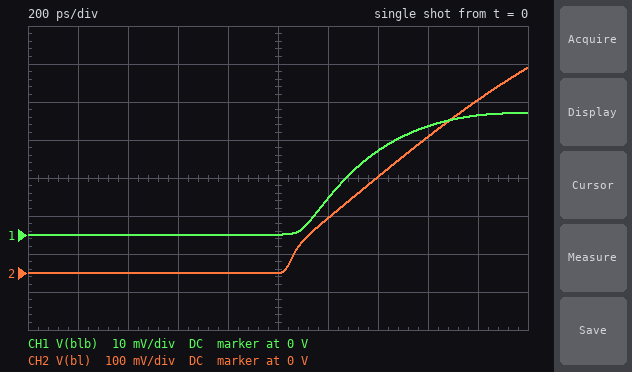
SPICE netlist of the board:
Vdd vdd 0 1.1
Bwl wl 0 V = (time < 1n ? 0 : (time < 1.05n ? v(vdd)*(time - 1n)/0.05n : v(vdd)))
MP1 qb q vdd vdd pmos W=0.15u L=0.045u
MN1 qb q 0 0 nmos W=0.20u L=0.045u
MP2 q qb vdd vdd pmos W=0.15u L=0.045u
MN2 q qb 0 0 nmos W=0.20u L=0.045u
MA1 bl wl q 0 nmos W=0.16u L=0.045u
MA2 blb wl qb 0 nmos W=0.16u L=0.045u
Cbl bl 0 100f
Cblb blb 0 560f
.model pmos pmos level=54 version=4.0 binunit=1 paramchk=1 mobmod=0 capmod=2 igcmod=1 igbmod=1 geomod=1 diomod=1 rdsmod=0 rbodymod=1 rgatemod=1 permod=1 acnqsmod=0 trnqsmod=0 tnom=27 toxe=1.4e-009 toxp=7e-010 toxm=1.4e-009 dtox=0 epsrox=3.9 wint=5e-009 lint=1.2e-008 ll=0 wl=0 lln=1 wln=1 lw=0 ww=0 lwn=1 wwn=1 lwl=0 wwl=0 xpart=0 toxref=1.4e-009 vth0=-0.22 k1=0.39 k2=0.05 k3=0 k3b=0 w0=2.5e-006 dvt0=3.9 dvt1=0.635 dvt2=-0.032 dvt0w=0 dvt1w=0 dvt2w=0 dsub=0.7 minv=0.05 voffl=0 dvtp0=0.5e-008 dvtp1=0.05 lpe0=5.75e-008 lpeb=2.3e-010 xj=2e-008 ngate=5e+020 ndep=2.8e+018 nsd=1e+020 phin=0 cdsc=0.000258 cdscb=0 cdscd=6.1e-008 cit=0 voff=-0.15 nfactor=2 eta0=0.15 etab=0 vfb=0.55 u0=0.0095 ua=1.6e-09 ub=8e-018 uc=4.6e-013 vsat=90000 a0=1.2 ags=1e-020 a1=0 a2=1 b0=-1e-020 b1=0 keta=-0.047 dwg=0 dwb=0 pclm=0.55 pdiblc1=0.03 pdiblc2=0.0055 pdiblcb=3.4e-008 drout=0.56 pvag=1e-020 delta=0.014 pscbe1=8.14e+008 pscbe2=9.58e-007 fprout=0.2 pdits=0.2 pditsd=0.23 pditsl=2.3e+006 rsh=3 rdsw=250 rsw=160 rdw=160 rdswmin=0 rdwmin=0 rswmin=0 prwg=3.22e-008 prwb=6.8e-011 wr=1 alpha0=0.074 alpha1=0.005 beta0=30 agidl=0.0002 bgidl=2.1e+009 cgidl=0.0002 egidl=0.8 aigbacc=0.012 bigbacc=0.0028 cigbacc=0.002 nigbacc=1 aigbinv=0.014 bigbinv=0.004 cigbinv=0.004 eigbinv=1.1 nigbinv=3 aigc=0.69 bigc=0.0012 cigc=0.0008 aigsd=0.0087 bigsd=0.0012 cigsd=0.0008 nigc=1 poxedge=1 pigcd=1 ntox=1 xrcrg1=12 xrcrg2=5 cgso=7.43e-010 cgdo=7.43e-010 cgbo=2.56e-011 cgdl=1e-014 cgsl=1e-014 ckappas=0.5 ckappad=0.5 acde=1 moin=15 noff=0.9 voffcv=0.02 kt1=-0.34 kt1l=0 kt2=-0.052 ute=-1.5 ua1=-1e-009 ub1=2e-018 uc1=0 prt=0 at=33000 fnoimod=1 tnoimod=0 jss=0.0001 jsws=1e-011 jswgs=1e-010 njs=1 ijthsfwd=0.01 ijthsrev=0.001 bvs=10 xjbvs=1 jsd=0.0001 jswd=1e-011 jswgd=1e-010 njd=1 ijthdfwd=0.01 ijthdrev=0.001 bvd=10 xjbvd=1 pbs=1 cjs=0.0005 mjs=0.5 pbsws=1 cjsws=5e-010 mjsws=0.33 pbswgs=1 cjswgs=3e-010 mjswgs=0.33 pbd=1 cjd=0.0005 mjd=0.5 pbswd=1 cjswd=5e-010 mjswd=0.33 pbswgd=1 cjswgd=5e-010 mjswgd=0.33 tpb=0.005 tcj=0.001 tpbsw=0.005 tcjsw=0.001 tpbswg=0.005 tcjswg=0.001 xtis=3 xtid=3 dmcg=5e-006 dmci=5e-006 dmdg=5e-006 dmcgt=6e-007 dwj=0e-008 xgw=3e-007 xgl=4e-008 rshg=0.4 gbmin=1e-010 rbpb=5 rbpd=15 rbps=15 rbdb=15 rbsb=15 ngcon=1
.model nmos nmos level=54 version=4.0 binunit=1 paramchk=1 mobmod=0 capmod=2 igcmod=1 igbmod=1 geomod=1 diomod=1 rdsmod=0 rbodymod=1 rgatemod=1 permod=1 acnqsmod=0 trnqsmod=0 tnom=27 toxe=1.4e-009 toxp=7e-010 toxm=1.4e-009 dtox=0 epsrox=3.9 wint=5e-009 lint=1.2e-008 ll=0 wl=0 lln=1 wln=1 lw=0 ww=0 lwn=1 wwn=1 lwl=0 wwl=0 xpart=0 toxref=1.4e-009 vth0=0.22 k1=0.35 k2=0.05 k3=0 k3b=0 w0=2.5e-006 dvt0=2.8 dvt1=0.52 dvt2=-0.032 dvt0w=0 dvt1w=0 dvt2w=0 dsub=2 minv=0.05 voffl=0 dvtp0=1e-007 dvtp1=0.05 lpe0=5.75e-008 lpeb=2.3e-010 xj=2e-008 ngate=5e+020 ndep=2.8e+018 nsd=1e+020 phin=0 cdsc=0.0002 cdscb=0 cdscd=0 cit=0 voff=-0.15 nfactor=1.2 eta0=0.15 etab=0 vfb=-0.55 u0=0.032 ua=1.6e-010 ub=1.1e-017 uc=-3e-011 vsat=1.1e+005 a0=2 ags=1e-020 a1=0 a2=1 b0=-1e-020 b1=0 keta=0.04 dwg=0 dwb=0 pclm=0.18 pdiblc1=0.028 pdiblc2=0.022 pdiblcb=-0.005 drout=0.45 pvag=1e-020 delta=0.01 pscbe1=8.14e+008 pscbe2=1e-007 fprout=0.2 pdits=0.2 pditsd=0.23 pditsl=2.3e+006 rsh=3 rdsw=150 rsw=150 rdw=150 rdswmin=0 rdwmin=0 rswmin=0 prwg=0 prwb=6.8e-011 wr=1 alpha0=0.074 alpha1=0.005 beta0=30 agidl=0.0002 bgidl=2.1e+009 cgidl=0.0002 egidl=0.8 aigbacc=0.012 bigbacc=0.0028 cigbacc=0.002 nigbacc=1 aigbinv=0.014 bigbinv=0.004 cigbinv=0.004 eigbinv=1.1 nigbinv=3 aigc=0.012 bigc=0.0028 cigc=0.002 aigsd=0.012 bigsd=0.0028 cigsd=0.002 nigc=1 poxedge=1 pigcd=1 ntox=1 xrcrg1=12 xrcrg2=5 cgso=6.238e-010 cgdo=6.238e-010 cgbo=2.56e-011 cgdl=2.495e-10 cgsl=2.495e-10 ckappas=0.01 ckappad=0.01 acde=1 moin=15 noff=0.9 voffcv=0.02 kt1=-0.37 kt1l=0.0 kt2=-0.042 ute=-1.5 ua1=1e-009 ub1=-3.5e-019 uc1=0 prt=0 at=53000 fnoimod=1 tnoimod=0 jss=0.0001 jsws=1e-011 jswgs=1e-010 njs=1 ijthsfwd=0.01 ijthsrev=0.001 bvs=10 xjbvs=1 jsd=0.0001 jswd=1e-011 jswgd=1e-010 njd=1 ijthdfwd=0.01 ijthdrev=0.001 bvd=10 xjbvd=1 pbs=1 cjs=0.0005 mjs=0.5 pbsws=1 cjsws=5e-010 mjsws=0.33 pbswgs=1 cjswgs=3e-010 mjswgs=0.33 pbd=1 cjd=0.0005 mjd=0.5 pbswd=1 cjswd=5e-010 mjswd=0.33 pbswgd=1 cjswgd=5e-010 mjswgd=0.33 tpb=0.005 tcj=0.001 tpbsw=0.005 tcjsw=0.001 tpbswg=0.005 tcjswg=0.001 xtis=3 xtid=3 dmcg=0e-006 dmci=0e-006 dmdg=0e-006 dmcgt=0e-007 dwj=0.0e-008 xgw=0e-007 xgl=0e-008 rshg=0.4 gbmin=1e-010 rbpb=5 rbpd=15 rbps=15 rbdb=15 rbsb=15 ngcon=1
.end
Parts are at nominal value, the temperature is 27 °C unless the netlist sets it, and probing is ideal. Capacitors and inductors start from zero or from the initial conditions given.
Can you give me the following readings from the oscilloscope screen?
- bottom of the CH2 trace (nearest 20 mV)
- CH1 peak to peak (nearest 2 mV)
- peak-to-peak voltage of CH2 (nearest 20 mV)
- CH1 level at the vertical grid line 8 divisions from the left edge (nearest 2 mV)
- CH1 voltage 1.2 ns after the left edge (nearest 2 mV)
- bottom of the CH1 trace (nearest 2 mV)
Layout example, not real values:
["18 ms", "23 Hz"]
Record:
["0 V", "32 mV", "540 mV", "28 mV", "10 mV", "0 V"]
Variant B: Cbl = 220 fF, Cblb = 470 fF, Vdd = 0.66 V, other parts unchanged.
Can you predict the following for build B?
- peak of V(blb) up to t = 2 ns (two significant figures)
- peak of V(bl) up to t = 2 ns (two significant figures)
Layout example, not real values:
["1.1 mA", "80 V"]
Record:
["33 mV", "110 mV"]
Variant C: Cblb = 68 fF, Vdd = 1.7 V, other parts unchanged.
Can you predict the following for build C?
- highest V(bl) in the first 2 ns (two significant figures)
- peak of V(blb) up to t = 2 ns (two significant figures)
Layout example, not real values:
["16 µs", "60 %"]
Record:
["140 mV", "1.1 V"]
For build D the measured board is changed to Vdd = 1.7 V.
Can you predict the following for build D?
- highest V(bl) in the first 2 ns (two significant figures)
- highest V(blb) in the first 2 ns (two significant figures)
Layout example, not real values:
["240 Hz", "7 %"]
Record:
["890 mV", "59 mV"]
